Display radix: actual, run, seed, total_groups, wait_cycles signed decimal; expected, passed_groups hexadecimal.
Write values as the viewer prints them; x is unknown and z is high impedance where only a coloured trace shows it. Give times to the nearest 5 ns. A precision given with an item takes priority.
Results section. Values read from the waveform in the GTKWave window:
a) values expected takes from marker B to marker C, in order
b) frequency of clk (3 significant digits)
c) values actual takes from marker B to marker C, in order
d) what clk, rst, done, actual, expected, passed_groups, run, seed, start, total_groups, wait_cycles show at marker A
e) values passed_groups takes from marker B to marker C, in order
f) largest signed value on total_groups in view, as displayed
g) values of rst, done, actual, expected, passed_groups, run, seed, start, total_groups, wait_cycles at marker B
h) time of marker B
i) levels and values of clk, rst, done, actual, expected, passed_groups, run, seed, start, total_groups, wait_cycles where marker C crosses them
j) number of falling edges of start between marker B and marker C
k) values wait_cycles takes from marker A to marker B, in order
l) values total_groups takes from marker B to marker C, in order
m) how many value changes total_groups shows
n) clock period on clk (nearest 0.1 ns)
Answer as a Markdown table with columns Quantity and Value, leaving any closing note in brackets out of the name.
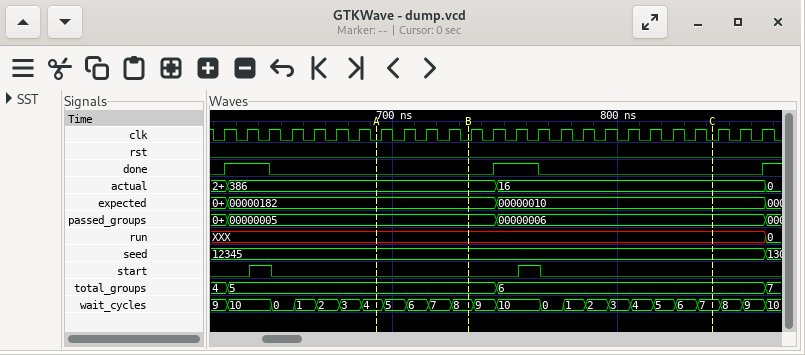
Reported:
| Quantity | Value |
|---|---|
| values expected takes from marker B to marker C, in order | 00000182, 00000010 |
| frequency of clk | 100 MHz |
| values actual takes from marker B to marker C, in order | 386, 16 |
| what clk, rst, done, actual, expected, passed_groups, run, seed, start, total_groups, wait_cycles show at marker A | clk=0, rst=0, done=0, actual=386, expected=00000182, passed_groups=00000005, run=XXX, seed=12345, start=0, total_groups=5, wait_cycles=4 |
| values passed_groups takes from marker B to marker C, in order | 00000005, 00000006 |
| largest signed value on total_groups in view, as displayed | 7 |
| values of rst, done, actual, expected, passed_groups, run, seed, start, total_groups, wait_cycles at marker B | rst=0, done=0, actual=386, expected=00000182, passed_groups=00000005, run=XXX, seed=12345, start=0, total_groups=5, wait_cycles=8 |
| time of marker B | 735 ns |
| levels and values of clk, rst, done, actual, expected, passed_groups, run, seed, start, total_groups, wait_cycles where marker C crosses them | clk=0, rst=0, done=0, actual=16, expected=00000010, passed_groups=00000006, run=XXX, seed=12345, start=0, total_groups=6, wait_cycles=7 |
| number of falling edges of start between marker B and marker C | 1 |
| values wait_cycles takes from marker A to marker B, in order | 4, 5, 6, 7, 8 |
| values total_groups takes from marker B to marker C, in order | 5, 6 |
| how many value changes total_groups shows | 3 |
| clock period on clk | 10 ns |
